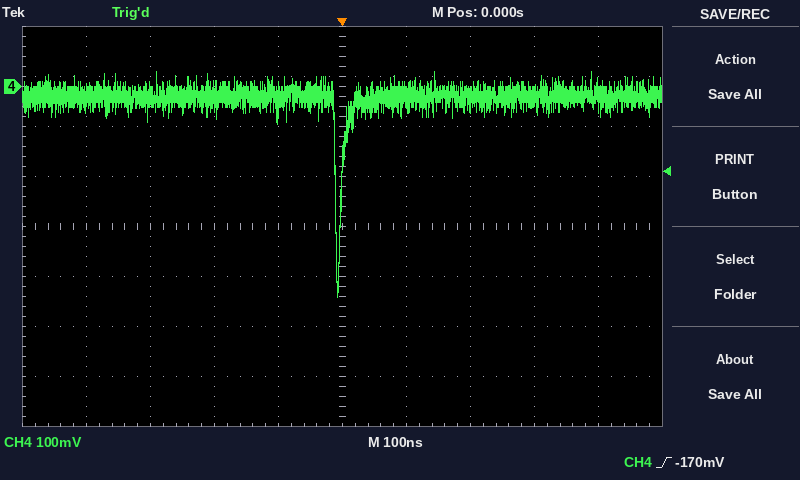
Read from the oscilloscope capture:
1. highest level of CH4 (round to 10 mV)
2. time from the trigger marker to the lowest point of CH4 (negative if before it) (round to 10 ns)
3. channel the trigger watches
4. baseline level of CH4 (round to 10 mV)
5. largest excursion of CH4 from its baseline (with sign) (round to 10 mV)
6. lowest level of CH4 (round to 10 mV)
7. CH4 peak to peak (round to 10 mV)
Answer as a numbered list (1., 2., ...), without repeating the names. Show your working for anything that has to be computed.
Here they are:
1. 30 mV
2. -10 ns
3. CH4
4. -20 mV
5. -420 mV − (-20 mV) = -400 mV
6. -420 mV
7. 30 mV − (-420 mV) = 450 mV
